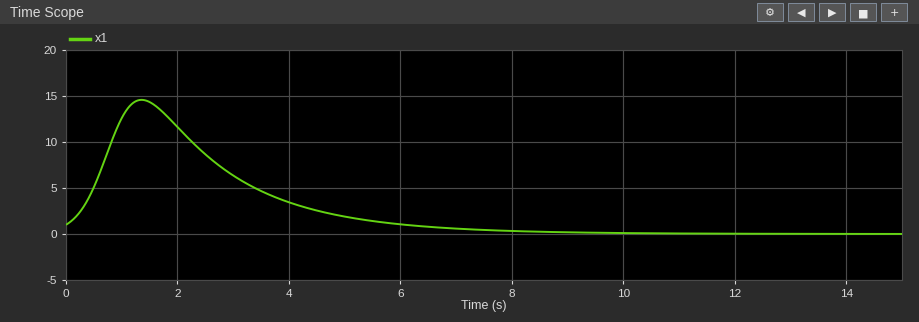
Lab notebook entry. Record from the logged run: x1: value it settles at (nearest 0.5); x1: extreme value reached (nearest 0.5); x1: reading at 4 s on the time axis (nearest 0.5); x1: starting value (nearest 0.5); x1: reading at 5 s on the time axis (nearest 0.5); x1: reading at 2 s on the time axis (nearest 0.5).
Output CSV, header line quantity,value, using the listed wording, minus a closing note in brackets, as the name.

quantity,value
x1: value it settles at,0.0
x1: extreme value reached,14.5
x1: reading at 4 s on the time axis,3.5
x1: starting value,1.0
x1: reading at 5 s on the time axis,2.0
x1: reading at 2 s on the time axis,11.5
